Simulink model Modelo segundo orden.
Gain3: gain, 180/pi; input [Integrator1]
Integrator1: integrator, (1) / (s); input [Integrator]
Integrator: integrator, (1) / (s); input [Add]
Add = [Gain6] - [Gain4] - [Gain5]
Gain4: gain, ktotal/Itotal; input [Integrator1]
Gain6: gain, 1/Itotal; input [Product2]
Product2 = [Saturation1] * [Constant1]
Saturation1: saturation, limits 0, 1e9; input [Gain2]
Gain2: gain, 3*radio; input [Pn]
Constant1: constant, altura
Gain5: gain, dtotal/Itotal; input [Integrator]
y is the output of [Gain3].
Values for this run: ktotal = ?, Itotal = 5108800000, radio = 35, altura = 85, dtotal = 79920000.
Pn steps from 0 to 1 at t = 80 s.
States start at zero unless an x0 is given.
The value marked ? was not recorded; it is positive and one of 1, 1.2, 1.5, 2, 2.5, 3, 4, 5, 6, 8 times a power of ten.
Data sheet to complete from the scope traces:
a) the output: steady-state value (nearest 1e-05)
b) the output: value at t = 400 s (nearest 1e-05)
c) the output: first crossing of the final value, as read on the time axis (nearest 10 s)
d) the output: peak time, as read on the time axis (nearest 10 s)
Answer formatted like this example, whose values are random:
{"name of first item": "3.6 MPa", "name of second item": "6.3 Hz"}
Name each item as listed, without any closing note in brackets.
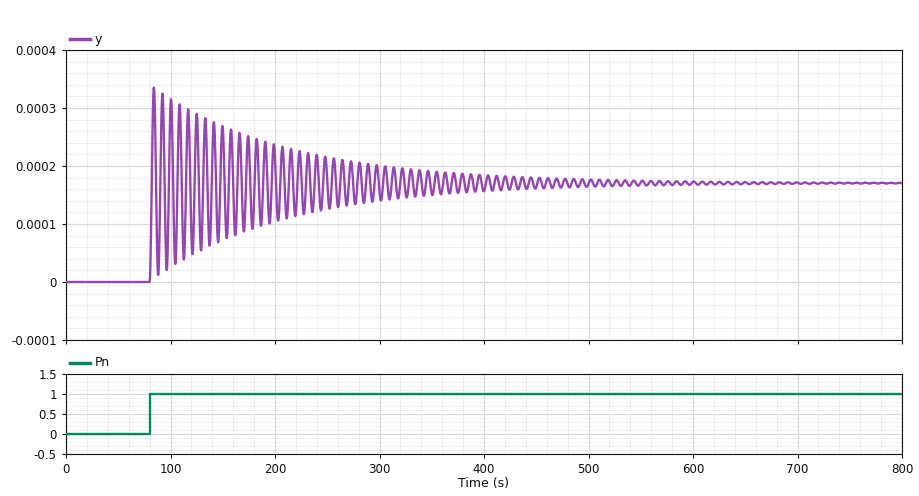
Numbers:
{"the output: steady-state value": "0.00017", "the output: value at t = 400 s": "0.00016", "the output: first crossing of the final value, as read on the time axis": "80 s", "the output: peak time, as read on the time axis": "80 s"}
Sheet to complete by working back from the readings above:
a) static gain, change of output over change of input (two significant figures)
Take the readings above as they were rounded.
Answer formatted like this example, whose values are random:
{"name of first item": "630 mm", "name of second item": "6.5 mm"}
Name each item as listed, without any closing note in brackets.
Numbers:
{"static gain, change of output over change of input": "0.00017"}
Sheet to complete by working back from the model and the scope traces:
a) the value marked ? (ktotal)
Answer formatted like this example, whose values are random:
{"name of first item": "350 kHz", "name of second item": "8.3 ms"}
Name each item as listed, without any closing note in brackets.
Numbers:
{"the value marked ?": "3e+09"}
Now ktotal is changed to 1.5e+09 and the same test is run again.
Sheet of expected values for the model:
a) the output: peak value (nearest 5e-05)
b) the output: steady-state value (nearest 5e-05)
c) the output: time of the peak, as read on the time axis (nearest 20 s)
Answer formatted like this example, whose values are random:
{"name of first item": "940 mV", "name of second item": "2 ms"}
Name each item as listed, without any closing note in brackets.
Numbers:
{"the output: peak value": "0.00065", "the output: steady-state value": "0.00035", "the output: time of the peak, as read on the time axis": "80 s"}
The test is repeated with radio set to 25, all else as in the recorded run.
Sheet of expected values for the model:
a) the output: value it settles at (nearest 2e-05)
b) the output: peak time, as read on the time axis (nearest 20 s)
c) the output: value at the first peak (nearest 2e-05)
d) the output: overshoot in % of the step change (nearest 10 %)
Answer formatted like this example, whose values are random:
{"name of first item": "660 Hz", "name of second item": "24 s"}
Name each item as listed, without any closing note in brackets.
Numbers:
{"the output: value it settles at": "0.00012", "the output: peak time, as read on the time axis": "80 s", "the output: value at the first peak": "0.00024", "the output: overshoot in % of the step change": "100 %"}
